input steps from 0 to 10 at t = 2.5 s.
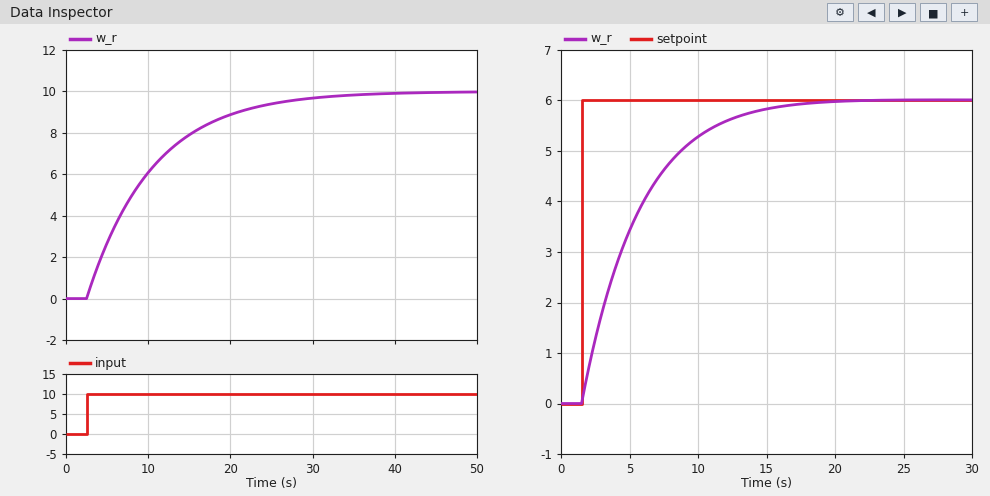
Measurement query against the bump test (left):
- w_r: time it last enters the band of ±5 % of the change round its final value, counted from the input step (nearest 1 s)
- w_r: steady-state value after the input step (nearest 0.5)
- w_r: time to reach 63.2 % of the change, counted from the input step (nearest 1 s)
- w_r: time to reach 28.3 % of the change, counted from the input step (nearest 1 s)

24 s
10.0
8 s
3 s
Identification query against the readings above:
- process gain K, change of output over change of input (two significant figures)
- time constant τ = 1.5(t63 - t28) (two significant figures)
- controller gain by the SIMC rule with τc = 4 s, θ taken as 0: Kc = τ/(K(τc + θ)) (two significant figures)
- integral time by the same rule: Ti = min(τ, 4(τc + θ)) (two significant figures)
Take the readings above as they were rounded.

1.0
7.5 s
1.9
7.5 s
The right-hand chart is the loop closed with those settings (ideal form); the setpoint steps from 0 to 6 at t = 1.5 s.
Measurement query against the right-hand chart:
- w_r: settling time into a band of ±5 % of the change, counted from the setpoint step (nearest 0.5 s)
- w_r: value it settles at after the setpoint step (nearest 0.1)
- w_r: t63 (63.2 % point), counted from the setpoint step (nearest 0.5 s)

11.5 s
6.0
4.0 s
